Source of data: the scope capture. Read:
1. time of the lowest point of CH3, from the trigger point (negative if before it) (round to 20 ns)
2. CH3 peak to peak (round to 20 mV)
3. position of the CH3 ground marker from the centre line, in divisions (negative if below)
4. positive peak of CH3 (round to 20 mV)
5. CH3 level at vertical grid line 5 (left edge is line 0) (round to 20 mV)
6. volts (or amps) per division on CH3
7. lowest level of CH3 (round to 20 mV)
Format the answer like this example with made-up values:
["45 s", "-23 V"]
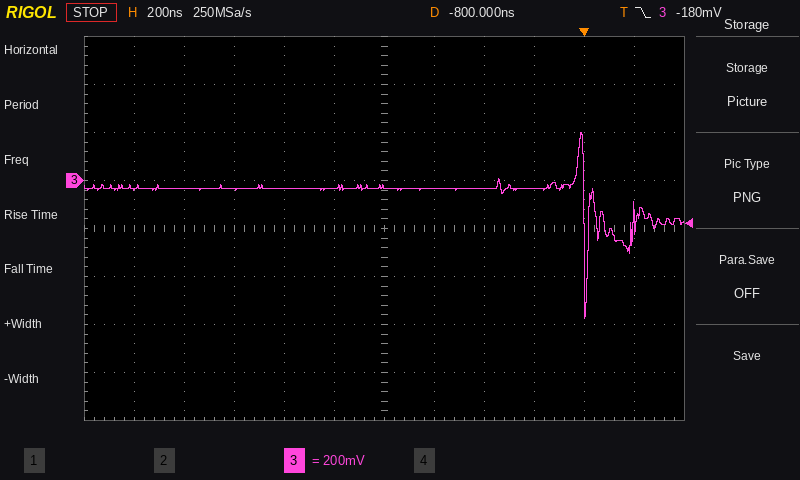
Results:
["0 ns", "780 mV", "+1.0 div", "200 mV", "-40 mV", "200 mV", "-580 mV"]
